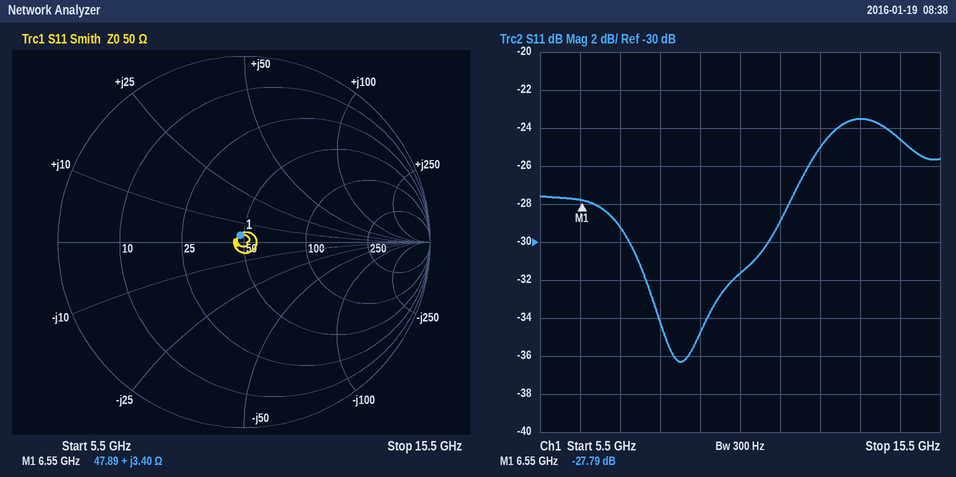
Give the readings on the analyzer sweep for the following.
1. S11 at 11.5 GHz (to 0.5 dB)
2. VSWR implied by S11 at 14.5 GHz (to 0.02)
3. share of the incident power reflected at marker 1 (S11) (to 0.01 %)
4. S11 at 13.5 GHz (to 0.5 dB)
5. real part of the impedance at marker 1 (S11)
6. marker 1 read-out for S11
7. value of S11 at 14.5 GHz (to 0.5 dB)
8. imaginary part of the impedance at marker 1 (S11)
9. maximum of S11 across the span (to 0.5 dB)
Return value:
-29.0 dB
1.12
0.17 %
-23.5 dB
47.89 Ω
-27.79 dB
-24.5 dB
+3.40 Ω
-23.5 dB
